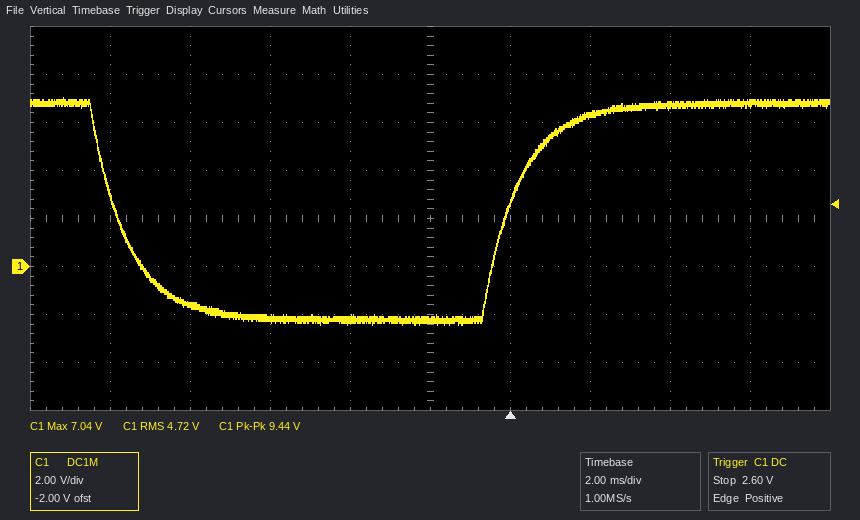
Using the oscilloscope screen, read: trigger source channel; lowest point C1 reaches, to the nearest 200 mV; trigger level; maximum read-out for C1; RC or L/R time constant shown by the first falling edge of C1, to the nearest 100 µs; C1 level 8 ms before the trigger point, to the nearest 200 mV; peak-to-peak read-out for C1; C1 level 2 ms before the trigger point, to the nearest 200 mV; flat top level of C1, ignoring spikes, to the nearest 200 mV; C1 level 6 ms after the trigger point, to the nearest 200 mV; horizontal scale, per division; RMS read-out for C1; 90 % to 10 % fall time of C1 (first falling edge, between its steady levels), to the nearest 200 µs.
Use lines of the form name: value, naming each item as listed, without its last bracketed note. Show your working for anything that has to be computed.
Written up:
trigger source channel: C1
lowest point C1 reaches, to the nearest 200 mV: -2.4 V
trigger level: 2.60 V
maximum read-out for C1: 7.04 V
RC or L/R time constant shown by the first falling edge of C1, to the nearest 100 µs: 2.0 ms / 2.2 ≈ 909 µs, so 900 µs to the nearest 100 µs
C1 level 8 ms before the trigger point, to the nearest 200 mV: -1.6 V
peak-to-peak read-out for C1: 9.44 V
C1 level 2 ms before the trigger point, to the nearest 200 mV: -2.2 V
flat top level of C1, ignoring spikes, to the nearest 200 mV: 6.8 V
C1 level 6 ms after the trigger point, to the nearest 200 mV: 6.8 V
horizontal scale, per division: 2 ms
RMS read-out for C1: 4.72 V
90 % to 10 % fall time of C1 (first falling edge, between its steady levels), to the nearest 200 µs: 2.0 ms
